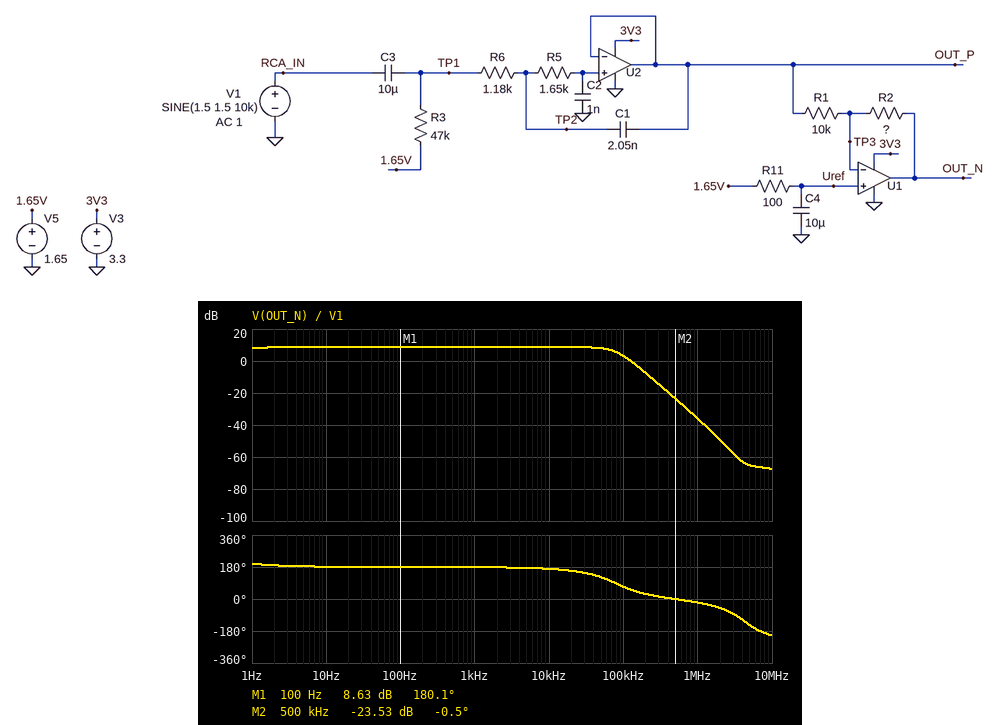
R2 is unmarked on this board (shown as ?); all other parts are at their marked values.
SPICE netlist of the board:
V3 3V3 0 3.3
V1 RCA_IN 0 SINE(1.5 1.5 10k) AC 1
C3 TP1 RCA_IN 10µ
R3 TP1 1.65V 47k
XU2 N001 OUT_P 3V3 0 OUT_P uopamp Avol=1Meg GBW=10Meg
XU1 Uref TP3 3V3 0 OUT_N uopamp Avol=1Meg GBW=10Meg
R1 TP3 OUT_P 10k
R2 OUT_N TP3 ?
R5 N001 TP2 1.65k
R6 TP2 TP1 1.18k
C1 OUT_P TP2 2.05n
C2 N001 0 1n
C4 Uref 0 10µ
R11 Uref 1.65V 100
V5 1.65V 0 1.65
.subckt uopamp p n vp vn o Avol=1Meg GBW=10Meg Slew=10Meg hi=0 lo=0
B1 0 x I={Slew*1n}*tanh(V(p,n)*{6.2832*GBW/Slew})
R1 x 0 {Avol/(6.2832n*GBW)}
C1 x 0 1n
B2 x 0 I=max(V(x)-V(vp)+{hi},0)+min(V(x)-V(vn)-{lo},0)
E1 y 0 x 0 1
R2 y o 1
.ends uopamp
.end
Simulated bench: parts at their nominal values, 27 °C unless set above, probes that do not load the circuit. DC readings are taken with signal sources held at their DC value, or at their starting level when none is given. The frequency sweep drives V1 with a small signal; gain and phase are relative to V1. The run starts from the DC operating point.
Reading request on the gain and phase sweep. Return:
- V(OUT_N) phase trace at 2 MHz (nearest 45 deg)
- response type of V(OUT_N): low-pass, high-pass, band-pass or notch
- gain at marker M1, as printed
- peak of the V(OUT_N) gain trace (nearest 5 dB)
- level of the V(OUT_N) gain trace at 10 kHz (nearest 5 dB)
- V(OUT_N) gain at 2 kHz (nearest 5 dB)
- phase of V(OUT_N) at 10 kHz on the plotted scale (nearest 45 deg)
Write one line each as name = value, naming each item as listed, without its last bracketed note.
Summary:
V(OUT_N) phase trace at 2 MHz = -45 deg
response type of V(OUT_N): low-pass, high-pass, band-pass or notch = low-pass
gain at marker M1, as printed = 8.63 dB
peak of the V(OUT_N) gain trace = 10 dB
level of the V(OUT_N) gain trace at 10 kHz = 10 dB
V(OUT_N) gain at 2 kHz = 10 dB
phase of V(OUT_N) at 10 kHz on the plotted scale = 180 deg
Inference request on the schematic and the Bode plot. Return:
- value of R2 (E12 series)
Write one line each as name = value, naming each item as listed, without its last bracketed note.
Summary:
value of R2 = 27 kΩ
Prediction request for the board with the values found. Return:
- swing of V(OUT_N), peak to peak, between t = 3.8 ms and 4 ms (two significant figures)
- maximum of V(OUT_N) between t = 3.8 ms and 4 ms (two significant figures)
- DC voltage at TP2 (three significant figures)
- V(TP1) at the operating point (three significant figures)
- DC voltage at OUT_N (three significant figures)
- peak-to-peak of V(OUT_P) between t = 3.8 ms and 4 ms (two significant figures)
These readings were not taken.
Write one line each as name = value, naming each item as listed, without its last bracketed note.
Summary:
swing of V(OUT_N), peak to peak, between t = 3.8 ms and 4 ms = 3.3 V
maximum of V(OUT_N) between t = 3.8 ms and 4 ms = 3.3 V
DC voltage at TP2 = 1.65 V
V(TP1) at the operating point = 1.65 V
DC voltage at OUT_N = 1.65 V
peak-to-peak of V(OUT_P) between t = 3.8 ms and 4 ms = 3.0 V
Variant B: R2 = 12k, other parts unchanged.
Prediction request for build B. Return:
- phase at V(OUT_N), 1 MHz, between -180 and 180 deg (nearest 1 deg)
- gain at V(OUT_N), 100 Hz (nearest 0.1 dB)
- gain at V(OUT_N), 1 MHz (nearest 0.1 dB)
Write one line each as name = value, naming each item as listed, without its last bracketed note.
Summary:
phase at V(OUT_N), 1 MHz, between -180 and 180 deg = -12 deg
gain at V(OUT_N), 100 Hz = 1.6 dB
gain at V(OUT_N), 1 MHz = -42.7 dB
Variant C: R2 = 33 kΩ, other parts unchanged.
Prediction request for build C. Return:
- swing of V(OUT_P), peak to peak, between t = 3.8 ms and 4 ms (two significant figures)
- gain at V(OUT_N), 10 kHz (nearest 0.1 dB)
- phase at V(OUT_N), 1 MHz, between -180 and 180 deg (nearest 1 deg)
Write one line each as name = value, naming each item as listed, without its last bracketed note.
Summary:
swing of V(OUT_P), peak to peak, between t = 3.8 ms and 4 ms = 3.0 V
gain at V(OUT_N), 10 kHz = 10.4 dB
phase at V(OUT_N), 1 MHz, between -180 and 180 deg = -23 deg
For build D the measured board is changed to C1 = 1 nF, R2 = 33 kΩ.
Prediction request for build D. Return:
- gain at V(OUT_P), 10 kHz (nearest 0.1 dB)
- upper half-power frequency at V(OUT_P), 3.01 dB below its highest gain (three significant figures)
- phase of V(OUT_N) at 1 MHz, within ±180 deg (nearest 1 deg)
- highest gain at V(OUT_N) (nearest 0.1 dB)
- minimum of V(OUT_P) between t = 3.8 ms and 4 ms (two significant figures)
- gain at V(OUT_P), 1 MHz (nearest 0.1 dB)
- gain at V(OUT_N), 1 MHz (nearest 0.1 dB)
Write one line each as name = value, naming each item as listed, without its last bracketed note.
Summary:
gain at V(OUT_P), 10 kHz = -0.1 dB
upper half-power frequency at V(OUT_P), 3.01 dB below its highest gain = 72.1 kHz
phase of V(OUT_N) at 1 MHz, within ±180 deg = -16 deg
highest gain at V(OUT_N) = 10.4 dB
minimum of V(OUT_P) between t = 3.8 ms and 4 ms = 160 mV
gain at V(OUT_P), 1 MHz = -38.0 dB
gain at V(OUT_N), 1 MHz = -28.3 dB
